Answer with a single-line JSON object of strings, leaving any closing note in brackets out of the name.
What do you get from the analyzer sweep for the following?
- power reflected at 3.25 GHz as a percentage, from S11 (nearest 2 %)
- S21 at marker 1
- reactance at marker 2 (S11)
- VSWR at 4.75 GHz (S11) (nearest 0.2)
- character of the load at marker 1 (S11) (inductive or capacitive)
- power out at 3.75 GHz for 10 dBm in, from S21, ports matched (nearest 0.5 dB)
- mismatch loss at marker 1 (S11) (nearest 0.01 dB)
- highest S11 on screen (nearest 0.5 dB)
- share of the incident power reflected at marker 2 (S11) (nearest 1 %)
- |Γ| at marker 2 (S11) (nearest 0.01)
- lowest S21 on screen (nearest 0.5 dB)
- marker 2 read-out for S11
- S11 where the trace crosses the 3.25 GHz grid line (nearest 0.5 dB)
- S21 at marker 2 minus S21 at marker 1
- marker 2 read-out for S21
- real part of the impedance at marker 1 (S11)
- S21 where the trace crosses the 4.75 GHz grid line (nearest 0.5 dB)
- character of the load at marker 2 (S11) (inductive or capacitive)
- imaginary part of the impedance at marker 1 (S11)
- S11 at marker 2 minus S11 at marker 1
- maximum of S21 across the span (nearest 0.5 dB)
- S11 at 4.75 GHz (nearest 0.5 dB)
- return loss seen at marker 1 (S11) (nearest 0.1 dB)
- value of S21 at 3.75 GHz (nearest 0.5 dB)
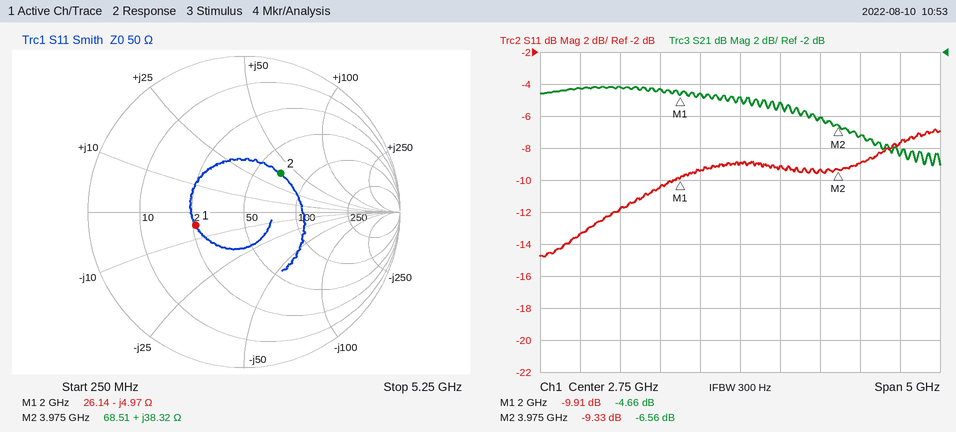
{"power reflected at 3.25 GHz as a percentage, from S11": "12 %", "S21 at marker 1": "-4.66 dB", "reactance at marker 2": "+38.32 Ω", "VSWR at 4.75 GHz (S11)": "2.4", "character of the load at marker 1 (S11)": "capacitive", "power out at 3.75 GHz for 10 dBm in, from S21, ports matched": "4.0 dBm", "mismatch loss at marker 1 (S11)": "0.47 dB", "highest S11 on screen": "-7.0 dB", "share of the incident power reflected at marker 2 (S11)": "12 %", "|Γ| at marker 2 (S11)": "0.34", "lowest S21 on screen": "-9.0 dB", "marker 2 read-out for S11": "-9.33 dB", "S11 where the trace crosses the 3.25 GHz grid line": "-9.0 dB", "S21 at marker 2 minus S21 at marker 1": "-1.90 dB", "marker 2 read-out for S21": "-6.56 dB", "real part of the impedance at marker 1": "26.14 Ω", "S21 where the trace crosses the 4.75 GHz grid line": "-8.5 dB", "character of the load at marker 2 (S11)": "inductive", "imaginary part of the impedance at marker 1": "-4.97 Ω", "S11 at marker 2 minus S11 at marker 1": "0.58 dB", "maximum of S21 across the span": "-4.0 dB", "S11 at 4.75 GHz": "-7.5 dB", "return loss seen at marker 1 (S11)": "9.9 dB", "value of S21 at 3.75 GHz": "-6.0 dB"}
